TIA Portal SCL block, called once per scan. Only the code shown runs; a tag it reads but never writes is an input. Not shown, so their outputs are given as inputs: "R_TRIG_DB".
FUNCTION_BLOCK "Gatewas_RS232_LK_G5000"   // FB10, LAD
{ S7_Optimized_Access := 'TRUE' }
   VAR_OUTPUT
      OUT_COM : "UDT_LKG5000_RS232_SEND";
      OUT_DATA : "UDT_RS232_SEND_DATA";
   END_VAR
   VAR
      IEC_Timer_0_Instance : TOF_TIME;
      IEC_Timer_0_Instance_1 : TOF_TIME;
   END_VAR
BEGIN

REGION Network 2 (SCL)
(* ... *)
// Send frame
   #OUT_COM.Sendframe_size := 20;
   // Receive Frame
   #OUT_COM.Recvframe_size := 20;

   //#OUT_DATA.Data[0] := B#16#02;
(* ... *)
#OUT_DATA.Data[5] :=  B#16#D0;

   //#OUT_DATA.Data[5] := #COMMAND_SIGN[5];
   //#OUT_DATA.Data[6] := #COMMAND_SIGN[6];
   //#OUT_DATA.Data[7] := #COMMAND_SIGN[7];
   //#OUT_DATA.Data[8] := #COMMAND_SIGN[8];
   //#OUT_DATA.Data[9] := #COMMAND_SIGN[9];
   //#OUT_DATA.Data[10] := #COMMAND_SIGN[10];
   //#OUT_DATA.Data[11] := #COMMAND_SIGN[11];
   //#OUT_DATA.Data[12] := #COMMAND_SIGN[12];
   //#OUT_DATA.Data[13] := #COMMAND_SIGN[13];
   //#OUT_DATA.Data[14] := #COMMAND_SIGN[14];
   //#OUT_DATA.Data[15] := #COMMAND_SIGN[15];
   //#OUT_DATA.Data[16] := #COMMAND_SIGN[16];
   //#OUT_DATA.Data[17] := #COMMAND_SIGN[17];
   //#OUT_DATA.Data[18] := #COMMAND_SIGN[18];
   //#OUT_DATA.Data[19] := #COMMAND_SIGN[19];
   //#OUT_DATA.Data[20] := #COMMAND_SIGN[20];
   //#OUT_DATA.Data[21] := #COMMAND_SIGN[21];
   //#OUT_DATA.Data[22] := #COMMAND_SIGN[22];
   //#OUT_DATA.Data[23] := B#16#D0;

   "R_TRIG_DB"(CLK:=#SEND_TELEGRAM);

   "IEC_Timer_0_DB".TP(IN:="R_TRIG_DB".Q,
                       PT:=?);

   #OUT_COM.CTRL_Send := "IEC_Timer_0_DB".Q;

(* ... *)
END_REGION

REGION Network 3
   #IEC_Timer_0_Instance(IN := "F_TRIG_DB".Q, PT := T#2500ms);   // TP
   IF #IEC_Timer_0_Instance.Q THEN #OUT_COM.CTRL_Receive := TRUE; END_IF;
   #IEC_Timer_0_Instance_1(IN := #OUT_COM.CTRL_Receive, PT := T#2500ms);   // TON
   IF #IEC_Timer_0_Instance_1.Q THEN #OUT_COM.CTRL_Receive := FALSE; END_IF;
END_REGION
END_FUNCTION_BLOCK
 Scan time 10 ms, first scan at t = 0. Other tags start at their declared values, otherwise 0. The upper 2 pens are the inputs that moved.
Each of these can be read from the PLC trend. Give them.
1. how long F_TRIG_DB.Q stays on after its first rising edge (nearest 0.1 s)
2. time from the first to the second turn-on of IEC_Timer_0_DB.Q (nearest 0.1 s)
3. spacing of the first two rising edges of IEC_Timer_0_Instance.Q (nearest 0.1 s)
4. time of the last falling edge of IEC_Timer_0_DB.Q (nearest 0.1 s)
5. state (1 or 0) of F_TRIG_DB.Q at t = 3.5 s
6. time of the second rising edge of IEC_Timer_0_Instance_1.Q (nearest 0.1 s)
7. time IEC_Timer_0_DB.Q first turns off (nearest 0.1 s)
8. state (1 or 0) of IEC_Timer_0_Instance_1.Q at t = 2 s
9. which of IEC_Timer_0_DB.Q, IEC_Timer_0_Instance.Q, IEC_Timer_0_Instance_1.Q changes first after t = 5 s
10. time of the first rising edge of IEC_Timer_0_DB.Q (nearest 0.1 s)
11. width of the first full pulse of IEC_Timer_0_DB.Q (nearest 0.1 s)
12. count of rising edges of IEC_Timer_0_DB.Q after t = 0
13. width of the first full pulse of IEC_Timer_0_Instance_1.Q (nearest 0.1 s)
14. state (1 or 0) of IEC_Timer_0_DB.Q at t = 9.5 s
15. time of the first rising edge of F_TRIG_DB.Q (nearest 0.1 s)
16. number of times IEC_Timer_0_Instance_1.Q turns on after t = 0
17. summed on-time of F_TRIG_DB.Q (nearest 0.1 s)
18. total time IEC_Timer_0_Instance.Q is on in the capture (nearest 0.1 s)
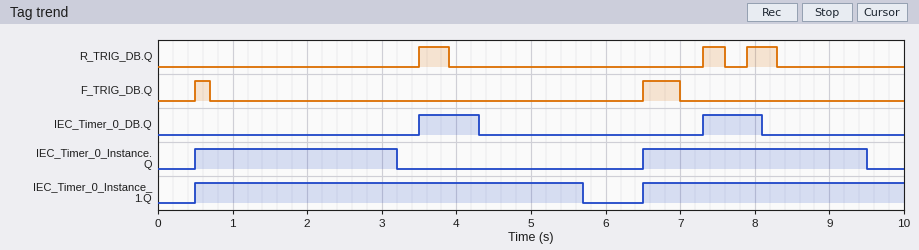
0.2 s
3.8 s
6.0 s
8.1 s
0
6.5 s
4.3 s
1
IEC_Timer_0_Instance_1.Q
3.5 s
0.8 s
2
5.2 s
0
0.5 s
2
0.7 s
5.7 s
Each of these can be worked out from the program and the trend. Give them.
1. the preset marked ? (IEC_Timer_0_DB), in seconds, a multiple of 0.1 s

0.8 s
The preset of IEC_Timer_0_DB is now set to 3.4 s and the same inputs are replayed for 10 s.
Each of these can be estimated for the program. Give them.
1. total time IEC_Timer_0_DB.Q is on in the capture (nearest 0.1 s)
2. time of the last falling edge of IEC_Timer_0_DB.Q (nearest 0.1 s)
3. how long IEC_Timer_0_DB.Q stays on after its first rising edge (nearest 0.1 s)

6.1 s
6.9 s
3.4 s
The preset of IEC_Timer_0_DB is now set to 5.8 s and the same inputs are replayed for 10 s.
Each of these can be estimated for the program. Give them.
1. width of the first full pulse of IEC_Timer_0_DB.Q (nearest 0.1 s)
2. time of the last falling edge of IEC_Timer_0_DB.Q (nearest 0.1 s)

5.8 s
9.3 s
